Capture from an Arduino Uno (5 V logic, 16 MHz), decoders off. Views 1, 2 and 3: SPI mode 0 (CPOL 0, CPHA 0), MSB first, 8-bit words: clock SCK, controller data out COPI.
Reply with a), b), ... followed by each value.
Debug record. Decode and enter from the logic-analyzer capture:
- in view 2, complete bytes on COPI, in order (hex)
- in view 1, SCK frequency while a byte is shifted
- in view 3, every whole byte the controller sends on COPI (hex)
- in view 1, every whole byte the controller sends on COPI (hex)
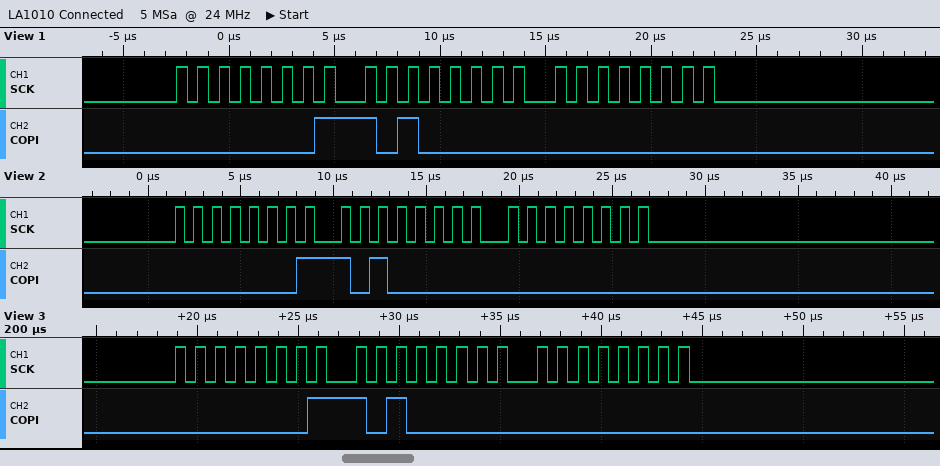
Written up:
a) 01 A0 00
b) 1 MHz
c) 0x01 0xA0 0x00
d) 0x01 0xA0 0x00
